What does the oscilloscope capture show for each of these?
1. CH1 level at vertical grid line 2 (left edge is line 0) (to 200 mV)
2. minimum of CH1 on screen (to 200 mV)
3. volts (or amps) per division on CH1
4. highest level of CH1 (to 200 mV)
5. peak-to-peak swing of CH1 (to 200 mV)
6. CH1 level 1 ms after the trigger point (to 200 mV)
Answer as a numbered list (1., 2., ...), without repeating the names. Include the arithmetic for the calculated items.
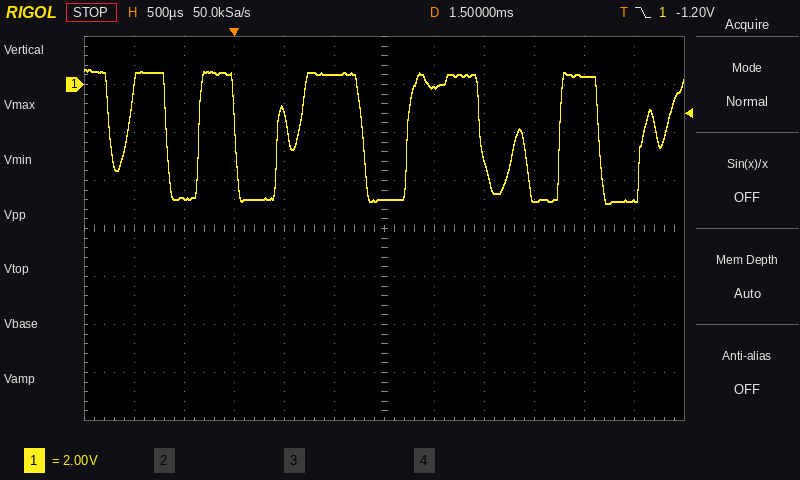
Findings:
1. -4.8 V
2. -5.0 V
3. 2 V
4. 600 mV
5. 600 mV − (-5.0 V) = 5.6 V
6. 400 mV
